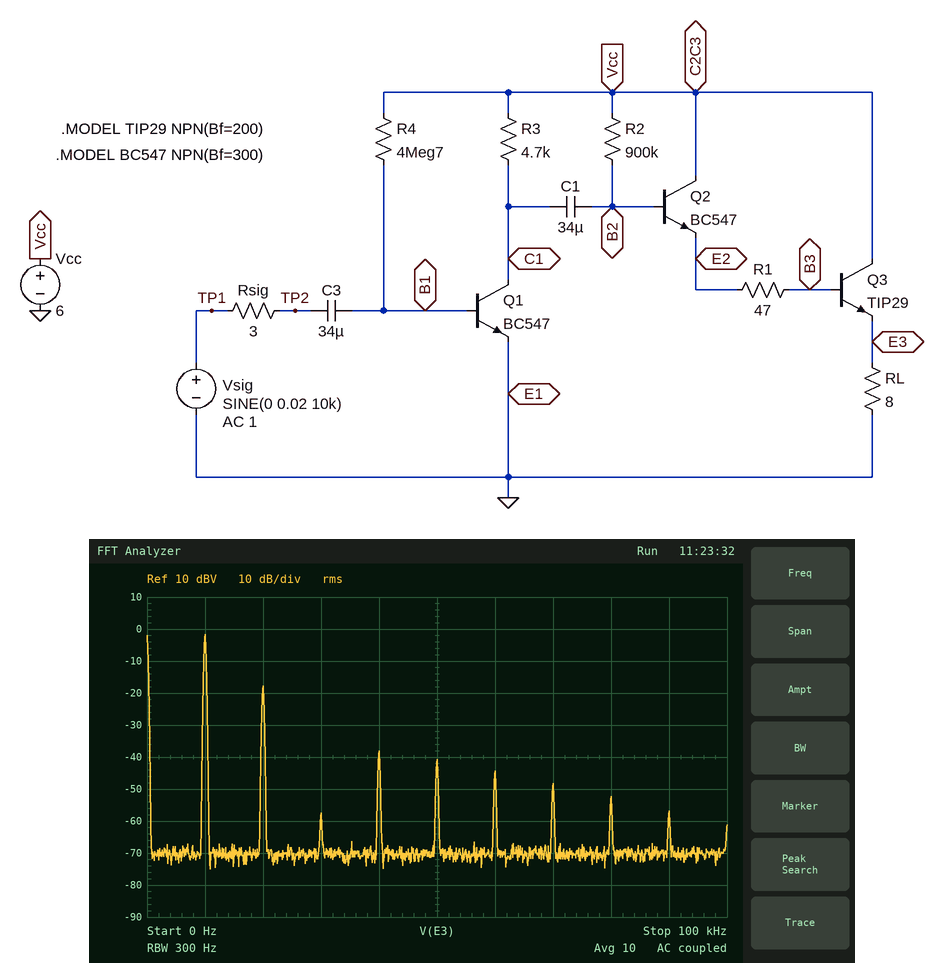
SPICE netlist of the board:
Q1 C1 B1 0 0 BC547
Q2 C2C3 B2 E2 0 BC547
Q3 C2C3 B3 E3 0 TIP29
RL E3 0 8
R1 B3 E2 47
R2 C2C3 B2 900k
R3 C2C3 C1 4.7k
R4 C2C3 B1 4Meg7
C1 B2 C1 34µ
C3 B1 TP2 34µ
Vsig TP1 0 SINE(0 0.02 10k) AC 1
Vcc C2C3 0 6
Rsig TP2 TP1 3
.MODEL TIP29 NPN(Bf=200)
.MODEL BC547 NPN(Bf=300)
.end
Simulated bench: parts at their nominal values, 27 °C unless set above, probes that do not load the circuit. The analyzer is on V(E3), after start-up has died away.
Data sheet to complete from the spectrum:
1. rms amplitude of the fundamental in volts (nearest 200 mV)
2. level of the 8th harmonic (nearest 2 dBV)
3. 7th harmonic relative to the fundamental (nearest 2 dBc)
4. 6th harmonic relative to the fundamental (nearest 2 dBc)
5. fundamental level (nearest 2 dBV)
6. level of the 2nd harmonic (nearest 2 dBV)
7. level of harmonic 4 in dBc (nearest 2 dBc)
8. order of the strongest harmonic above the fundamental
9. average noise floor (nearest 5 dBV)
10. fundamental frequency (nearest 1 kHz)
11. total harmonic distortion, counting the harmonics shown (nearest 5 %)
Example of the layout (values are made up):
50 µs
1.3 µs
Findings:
800 mV
-52 dBV
-46 dBc
-42 dBc
-2 dBV
-18 dBV
-36 dBc
2
-70 dBV
10 kHz
15 %
